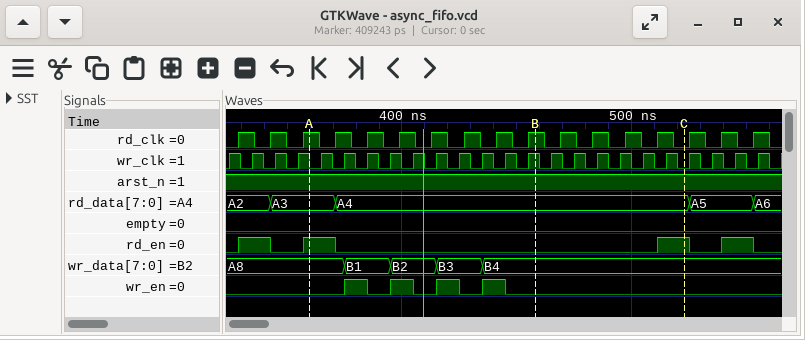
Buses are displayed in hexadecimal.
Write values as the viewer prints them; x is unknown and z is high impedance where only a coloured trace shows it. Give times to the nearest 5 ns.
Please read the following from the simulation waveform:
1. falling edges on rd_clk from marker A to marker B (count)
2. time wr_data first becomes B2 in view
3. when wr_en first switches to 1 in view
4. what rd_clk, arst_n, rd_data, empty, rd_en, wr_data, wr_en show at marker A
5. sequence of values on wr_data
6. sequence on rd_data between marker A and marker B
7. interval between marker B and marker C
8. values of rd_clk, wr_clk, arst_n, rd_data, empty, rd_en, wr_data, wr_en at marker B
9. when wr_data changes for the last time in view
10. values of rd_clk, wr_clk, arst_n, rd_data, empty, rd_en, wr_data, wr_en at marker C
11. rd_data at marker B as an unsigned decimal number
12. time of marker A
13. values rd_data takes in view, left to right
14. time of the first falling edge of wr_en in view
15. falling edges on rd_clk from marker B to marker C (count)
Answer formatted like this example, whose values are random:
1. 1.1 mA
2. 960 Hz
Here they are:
1. 7
2. 395 ns
3. 375 ns
4. rd_clk=1, arst_n=1, rd_data=A3, empty=0, rd_en=1, wr_data=A8, wr_en=0
5. A8, B1, B2, B3, B4
6. A3, A4
7. 65 ns
8. rd_clk=1, wr_clk=1, arst_n=1, rd_data=A4, empty=0, rd_en=0, wr_data=B4, wr_en=0
9. 435 ns
10. rd_clk=0, wr_clk=0, arst_n=1, rd_data=A4, empty=0, rd_en=1, wr_data=B4, wr_en=0
11. 164
12. 360 ns
13. A2, A3, A4, A5, A6
14. 385 ns
15. 5
